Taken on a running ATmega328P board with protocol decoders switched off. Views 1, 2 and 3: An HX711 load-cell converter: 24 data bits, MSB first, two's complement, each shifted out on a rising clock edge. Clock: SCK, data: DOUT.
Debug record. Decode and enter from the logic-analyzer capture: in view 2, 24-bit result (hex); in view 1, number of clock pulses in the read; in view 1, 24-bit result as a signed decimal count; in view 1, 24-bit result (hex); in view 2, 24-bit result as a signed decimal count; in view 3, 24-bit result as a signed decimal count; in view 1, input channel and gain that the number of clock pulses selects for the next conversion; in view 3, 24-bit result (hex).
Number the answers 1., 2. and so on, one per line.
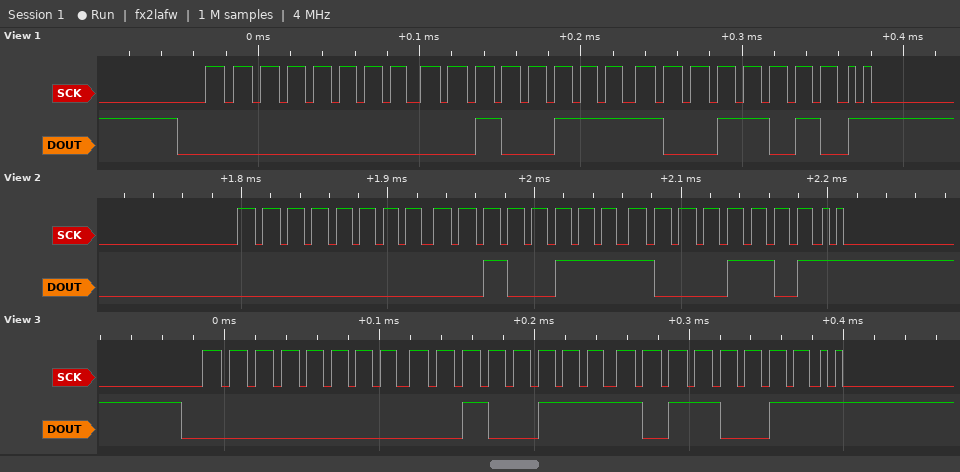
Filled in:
1. 0x00278D
2. 26
3. 10138
4. 0x00279A
5. 10125
6. 10163
7. channel B, gain 32
8. 0x0027B3
